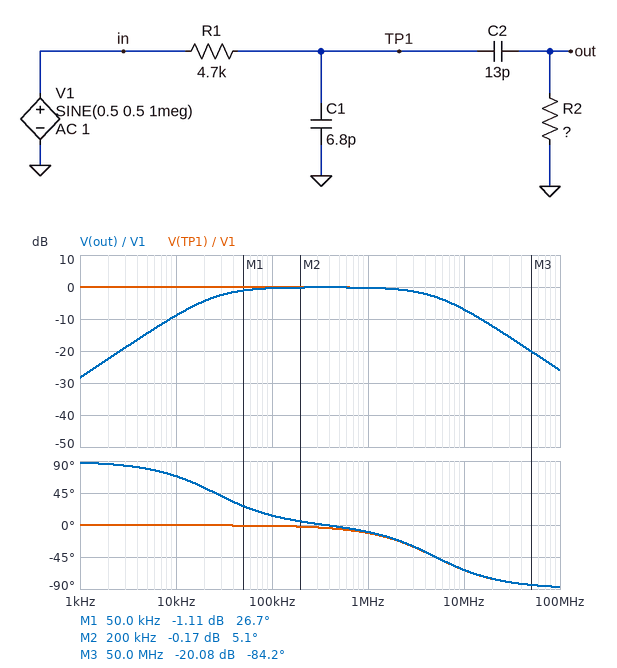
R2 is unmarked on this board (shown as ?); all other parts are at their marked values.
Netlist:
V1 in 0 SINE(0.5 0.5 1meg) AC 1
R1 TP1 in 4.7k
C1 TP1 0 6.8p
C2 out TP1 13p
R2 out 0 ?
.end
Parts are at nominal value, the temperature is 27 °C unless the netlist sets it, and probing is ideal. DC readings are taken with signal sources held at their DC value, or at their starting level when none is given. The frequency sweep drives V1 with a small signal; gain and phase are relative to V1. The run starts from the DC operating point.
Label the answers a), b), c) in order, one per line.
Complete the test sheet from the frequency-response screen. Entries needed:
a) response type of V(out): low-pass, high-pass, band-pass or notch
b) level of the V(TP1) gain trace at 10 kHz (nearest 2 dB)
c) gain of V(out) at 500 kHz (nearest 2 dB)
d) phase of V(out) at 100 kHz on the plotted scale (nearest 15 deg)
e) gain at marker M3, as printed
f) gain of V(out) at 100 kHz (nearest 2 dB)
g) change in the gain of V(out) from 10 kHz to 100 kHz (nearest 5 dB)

a) band-pass
b) 0 dB
c) 0 dB
d) 15 deg
e) -20.08 dB
f) 0 dB
g) 10 dB
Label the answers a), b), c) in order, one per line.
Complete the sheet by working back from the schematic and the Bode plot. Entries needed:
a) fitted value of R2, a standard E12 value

a) 470 kΩ
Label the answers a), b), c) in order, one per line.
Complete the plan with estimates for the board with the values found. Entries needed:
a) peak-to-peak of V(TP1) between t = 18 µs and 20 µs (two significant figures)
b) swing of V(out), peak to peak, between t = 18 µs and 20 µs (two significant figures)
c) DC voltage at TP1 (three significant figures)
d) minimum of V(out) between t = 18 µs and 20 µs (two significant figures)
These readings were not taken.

a) 970 mV
b) 970 mV
c) 500 mV
d) -490 mV
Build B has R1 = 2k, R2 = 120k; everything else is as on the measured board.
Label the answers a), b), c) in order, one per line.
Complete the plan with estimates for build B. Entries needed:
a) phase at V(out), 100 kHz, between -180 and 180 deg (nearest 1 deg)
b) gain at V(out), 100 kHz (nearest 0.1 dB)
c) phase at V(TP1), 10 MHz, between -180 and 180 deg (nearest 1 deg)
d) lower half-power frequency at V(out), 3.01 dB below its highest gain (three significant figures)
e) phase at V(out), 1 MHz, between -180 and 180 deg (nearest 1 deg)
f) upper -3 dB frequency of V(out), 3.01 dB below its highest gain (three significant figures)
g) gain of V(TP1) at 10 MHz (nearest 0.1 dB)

a) 45 deg
b) -3.2 dB
c) -40 deg
d) 98.7 kHz
e) 1 deg
f) 12.1 MHz
g) -2.5 dB
